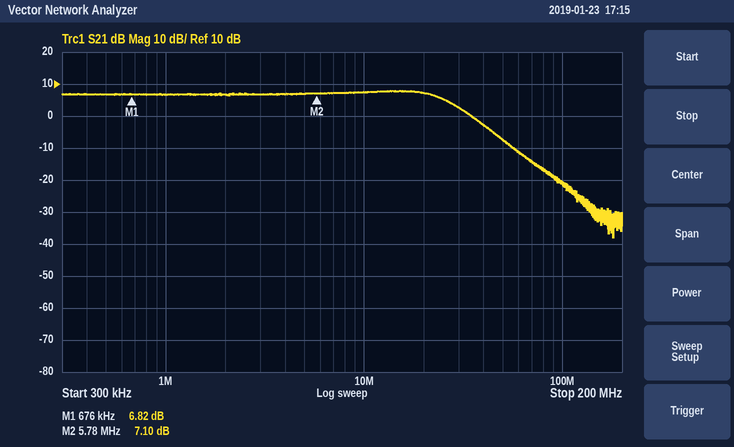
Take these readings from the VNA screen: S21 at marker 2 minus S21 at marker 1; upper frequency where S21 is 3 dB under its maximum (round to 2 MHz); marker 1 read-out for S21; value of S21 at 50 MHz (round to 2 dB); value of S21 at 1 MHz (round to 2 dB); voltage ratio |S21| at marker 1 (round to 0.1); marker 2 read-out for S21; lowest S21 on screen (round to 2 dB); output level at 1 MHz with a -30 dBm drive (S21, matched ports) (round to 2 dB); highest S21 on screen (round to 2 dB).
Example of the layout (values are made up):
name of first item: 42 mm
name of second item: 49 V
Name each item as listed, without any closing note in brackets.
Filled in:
S21 at marker 2 minus S21 at marker 1: 0.28 dB
upper frequency where S21 is 3 dB under its maximum: 26 MHz
marker 1 read-out for S21: 6.82 dB
value of S21 at 50 MHz: -8 dB
value of S21 at 1 MHz: 6 dB
voltage ratio |S21| at marker 1: 2.2
marker 2 read-out for S21: 7.10 dB
lowest S21 on screen: -38 dB
output level at 1 MHz with a -30 dBm drive (S21, matched ports): -24 dBm
highest S21 on screen: 8 dB
